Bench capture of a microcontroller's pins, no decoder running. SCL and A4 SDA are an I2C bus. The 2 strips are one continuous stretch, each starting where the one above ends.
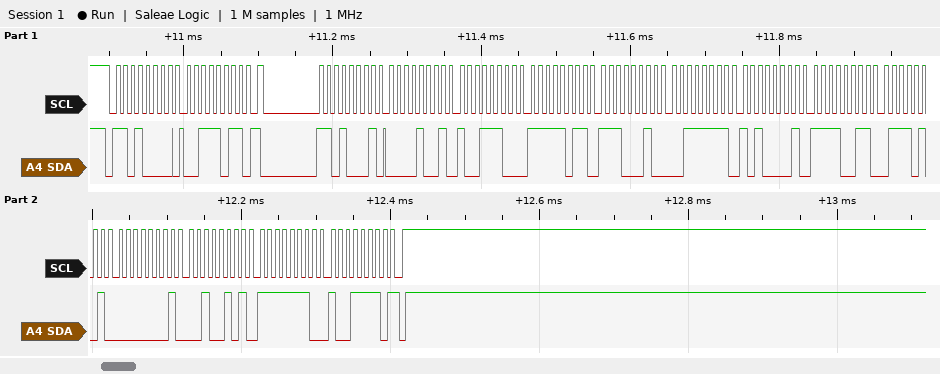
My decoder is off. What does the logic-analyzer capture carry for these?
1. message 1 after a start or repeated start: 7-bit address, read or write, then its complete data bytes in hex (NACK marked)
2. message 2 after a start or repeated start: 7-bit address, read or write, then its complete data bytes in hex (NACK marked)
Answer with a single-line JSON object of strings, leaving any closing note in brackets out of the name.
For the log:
{"message 1 after a start or repeated start: 7-bit address, read or write, then its complete data bytes in hex": "0x68 write: 3B", "message 2 after a start or repeated start: 7-bit address, read or write, then its complete data bytes in hex": "0x68 read: 09 9C FB E2 3F A1 F3 75 01 25 FE 9E NACK"}
